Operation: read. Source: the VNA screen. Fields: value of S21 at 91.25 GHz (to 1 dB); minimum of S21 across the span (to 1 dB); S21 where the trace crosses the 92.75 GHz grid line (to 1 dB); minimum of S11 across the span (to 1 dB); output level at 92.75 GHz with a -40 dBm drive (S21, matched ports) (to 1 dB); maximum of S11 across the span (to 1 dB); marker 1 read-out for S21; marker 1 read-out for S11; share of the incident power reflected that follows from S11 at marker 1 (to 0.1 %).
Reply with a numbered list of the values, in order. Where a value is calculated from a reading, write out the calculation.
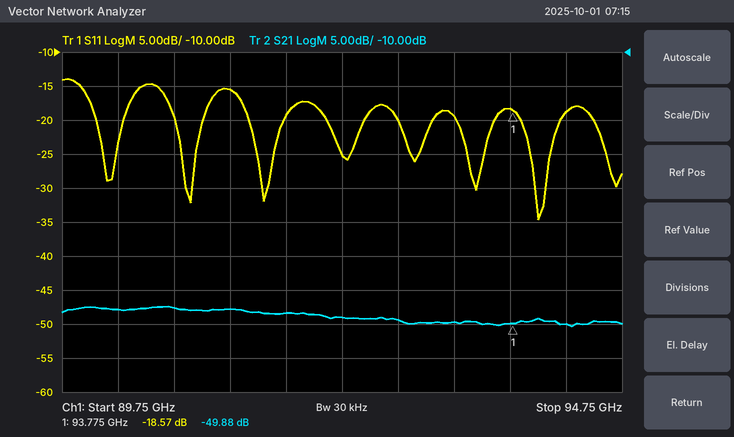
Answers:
1. -48 dB
2. -50 dB
3. -49 dB
4. -35 dB
5. -40 dBm + (-49 dB) = -89 dBm
6. -14 dB
7. -49.88 dB
8. -18.57 dB
9. 10^(-18.57/10) ≈ 1.4 %
